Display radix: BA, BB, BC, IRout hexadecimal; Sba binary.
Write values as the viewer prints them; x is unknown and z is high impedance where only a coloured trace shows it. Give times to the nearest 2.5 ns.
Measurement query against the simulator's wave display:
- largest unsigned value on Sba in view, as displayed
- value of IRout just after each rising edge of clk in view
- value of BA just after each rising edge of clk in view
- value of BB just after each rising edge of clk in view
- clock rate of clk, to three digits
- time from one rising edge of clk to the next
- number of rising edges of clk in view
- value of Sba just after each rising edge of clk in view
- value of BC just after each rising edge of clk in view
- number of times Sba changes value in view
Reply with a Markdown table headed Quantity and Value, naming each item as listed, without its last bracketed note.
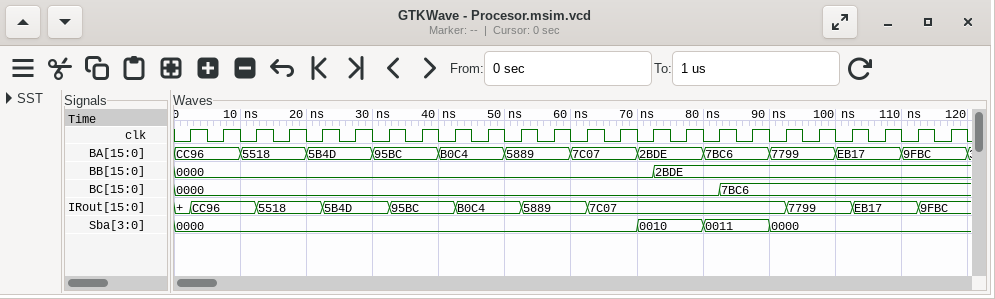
| Quantity | Value |
|---|---|
| largest unsigned value on Sba in view, as displayed | 0011 |
| value of IRout just after each rising edge of clk in view | CC96, CC96, 5518, 5518, 5B4D, 5B4D, 95BC, 95BC, B0C4, B0C4, 5889, 5889, 7C07, 7C07, 7C07, 7C07, 7C07, 7C07, 7799, 7799, EB17, EB17, 9FBC, 9FBC |
| value of BA just after each rising edge of clk in view | CC96, CC96, 5518, 5518, 5B4D, 5B4D, 95BC, 95BC, B0C4, B0C4, 5889, 5889, 7C07, 7C07, 2BDE, 2BDE, 7BC6, 7BC6, 7799, 7799, EB17, EB17, 9FBC, 9FBC |
| value of BB just after each rising edge of clk in view | 0000, 0000, 0000, 0000, 0000, 0000, 0000, 0000, 0000, 0000, 0000, 0000, 0000, 0000, 2BDE, 2BDE, 2BDE, 2BDE, 2BDE, 2BDE, 2BDE, 2BDE, 2BDE, 2BDE |
| clock rate of clk, to three digits | 200 MHz |
| time from one rising edge of clk to the next | 5 ns |
| number of rising edges of clk in view | 24 |
| value of Sba just after each rising edge of clk in view | 0000, 0000, 0000, 0000, 0000, 0000, 0000, 0000, 0000, 0000, 0000, 0000, 0000, 0000, 0010, 0010, 0011, 0011, 0000, 0000, 0000, 0000, 0000, 0000 |
| value of BC just after each rising edge of clk in view | 0000, 0000, 0000, 0000, 0000, 0000, 0000, 0000, 0000, 0000, 0000, 0000, 0000, 0000, 0000, 0000, 7BC6, 7BC6, 7BC6, 7BC6, 7BC6, 7BC6, 7BC6, 7BC6 |
| number of times Sba changes value in view | 3 |
